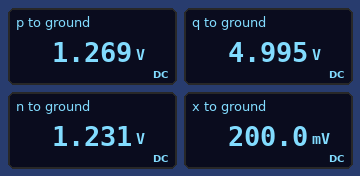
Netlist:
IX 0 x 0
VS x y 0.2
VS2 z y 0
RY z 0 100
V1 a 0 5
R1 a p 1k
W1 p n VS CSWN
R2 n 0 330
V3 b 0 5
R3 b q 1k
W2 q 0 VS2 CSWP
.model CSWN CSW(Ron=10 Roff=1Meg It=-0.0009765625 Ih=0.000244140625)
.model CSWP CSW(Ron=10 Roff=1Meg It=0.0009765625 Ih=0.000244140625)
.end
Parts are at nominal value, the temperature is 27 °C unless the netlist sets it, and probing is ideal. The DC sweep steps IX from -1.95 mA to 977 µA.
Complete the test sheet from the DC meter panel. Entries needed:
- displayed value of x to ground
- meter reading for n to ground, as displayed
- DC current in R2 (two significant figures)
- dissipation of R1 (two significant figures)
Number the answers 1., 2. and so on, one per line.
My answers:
1. 200.0 mV
2. 1.231 V
3. 3.7 mA
4. 14 mW
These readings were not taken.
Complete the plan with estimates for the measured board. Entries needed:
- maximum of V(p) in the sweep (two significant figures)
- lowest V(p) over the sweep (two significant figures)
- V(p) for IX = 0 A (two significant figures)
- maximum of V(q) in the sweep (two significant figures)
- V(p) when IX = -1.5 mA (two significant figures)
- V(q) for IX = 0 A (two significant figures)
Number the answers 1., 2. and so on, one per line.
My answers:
1. 5.0 V
2. 1.3 V
3. 1.3 V
4. 5.0 V
5. 5.0 V
6. 5.0 V
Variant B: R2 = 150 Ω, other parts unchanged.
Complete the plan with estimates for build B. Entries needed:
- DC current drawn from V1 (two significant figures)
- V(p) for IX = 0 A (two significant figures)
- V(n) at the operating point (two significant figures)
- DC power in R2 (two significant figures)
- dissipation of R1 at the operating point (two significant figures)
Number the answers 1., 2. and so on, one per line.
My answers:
1. 4.3 mA
2. 690 mV
3. 650 mV
4. 2.8 mW
5. 19 mW
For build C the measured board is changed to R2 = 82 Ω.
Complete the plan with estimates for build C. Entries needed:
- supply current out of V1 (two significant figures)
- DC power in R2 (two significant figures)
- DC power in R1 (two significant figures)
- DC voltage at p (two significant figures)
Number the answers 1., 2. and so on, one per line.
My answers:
1. 4.6 mA
2. 1.7 mW
3. 21 mW
4. 420 mV
